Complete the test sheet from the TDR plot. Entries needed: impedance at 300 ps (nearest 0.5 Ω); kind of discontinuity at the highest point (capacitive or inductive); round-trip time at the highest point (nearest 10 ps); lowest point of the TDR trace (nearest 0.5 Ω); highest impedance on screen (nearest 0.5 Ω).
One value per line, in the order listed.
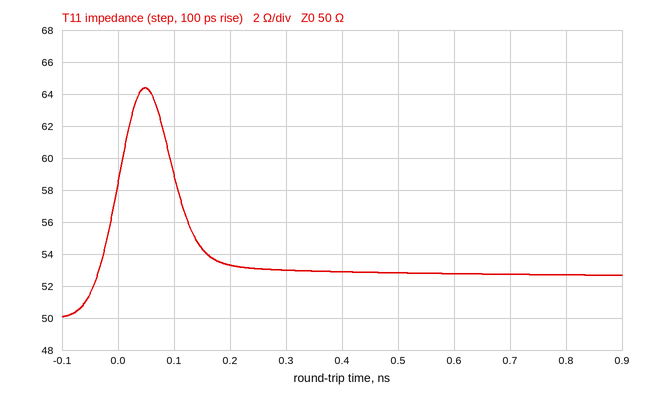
53.0 Ω
inductive
50 ps
50.0 Ω
64.5 Ω
